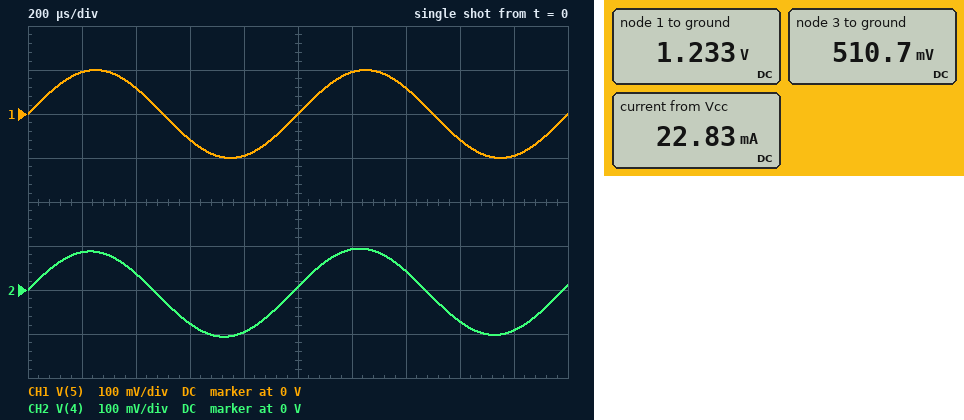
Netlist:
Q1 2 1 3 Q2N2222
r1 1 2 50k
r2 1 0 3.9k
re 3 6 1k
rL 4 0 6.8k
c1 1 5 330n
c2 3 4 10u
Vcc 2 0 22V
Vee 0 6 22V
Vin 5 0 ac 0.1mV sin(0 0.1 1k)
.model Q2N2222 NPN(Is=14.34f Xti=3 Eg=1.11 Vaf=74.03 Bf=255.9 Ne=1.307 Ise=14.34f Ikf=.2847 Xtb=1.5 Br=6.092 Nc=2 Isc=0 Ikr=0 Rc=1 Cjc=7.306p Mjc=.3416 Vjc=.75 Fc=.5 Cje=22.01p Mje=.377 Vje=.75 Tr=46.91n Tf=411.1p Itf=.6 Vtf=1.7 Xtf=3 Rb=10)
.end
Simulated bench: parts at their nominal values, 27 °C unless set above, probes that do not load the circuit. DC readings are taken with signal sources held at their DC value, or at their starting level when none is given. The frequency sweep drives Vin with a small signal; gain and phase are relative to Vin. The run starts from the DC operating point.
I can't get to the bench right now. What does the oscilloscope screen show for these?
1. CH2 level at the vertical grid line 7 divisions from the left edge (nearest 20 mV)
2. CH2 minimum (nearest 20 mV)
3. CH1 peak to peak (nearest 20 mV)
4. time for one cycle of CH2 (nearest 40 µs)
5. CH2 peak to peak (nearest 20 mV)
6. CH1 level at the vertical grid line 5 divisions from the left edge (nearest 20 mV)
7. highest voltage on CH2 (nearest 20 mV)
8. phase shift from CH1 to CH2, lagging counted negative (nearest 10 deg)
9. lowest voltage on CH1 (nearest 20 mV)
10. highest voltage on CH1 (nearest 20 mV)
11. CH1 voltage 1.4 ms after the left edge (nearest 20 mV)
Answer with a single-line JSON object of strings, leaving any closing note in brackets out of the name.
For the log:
{"CH2 level at the vertical grid line 7 divisions from the left edge": "40 mV", "CH2 minimum": "-100 mV", "CH1 peak to peak": "200 mV", "time for one cycle of CH2": "1.00 ms", "CH2 peak to peak": "200 mV", "CH1 level at the vertical grid line 5 divisions from the left edge": "0 V", "highest voltage on CH2": "100 mV", "phase shift from CH1 to CH2, lagging counted negative": "10 deg", "lowest voltage on CH1": "-100 mV", "highest voltage on CH1": "100 mV", "CH1 voltage 1.4 ms after the left edge": "60 mV"}
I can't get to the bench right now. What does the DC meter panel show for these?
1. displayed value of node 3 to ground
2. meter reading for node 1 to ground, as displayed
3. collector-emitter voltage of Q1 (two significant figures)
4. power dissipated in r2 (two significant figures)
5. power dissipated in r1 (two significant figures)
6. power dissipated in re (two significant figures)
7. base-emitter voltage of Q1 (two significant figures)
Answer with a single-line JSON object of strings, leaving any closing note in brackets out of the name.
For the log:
{"displayed value of node 3 to ground": "510.7 mV", "meter reading for node 1 to ground, as displayed": "1.233 V", "collector-emitter voltage of Q1": "21 V", "power dissipated in r2": "390 µW", "power dissipated in r1": "8.6 mW", "power dissipated in re": "510 mW", "base-emitter voltage of Q1": "720 mV"}
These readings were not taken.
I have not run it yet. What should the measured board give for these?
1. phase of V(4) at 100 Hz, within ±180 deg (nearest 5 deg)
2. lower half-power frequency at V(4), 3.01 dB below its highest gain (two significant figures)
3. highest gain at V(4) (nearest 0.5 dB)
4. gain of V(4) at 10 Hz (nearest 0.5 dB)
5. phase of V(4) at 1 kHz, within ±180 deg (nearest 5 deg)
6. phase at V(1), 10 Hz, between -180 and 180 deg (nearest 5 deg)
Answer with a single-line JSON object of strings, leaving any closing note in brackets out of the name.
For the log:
{"phase of V(4) at 100 Hz, within ±180 deg": "55 deg", "lower half-power frequency at V(4), 3.01 dB below its highest gain": "140 Hz", "highest gain at V(4)": "0 dB", "gain of V(4) at 10 Hz": "-23.0 dB", "phase of V(4) at 1 kHz, within ±180 deg": "10 deg", "phase at V(1), 10 Hz, between -180 and 180 deg": "85 deg"}
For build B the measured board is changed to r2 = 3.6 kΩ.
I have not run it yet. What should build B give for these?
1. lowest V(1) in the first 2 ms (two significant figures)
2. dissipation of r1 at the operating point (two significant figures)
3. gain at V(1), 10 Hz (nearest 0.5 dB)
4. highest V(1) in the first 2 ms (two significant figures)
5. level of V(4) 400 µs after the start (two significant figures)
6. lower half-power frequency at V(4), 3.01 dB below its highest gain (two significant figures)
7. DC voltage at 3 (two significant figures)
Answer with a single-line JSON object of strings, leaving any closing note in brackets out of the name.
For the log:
{"lowest V(1) in the first 2 ms": "1.0 V", "dissipation of r1 at the operating point": "8.7 mW", "gain at V(1), 10 Hz": "-23.5 dB", "highest V(1) in the first 2 ms": "1.2 V", "level of V(4) 400 µs after the start": "36 mV", "lower half-power frequency at V(4), 3.01 dB below its highest gain": "150 Hz", "DC voltage at 3": "420 mV"}
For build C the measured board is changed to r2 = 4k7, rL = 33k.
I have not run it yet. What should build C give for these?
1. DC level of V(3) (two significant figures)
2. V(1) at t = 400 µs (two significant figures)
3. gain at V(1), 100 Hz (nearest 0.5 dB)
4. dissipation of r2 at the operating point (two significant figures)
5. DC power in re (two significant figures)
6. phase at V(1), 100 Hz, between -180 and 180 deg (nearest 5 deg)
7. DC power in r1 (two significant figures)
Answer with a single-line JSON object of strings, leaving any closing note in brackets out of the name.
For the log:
{"DC level of V(3)": "740 mV", "V(1) at t = 400 µs": "1.5 V", "gain at V(1), 100 Hz": "-3.5 dB", "dissipation of r2 at the operating point": "450 µW", "DC power in re": "520 mW", "phase at V(1), 100 Hz, between -180 and 180 deg": "50 deg", "DC power in r1": "8.4 mW"}
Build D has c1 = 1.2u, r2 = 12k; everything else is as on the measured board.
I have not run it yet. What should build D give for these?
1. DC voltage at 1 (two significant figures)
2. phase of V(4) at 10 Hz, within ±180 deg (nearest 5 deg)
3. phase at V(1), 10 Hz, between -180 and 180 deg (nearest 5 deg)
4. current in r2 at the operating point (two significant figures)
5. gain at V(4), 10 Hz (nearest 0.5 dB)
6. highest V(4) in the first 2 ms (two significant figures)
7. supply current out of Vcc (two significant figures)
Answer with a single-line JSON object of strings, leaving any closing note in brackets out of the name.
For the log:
{"DC voltage at 1": "3.2 V", "phase of V(4) at 10 Hz, within ±180 deg": "70 deg", "phase at V(1), 10 Hz, between -180 and 180 deg": "55 deg", "current in r2 at the operating point": "270 µA", "gain at V(4), 10 Hz": "-5.0 dB", "highest V(4) in the first 2 ms": "98 mV", "supply current out of Vcc": "25 mA"}
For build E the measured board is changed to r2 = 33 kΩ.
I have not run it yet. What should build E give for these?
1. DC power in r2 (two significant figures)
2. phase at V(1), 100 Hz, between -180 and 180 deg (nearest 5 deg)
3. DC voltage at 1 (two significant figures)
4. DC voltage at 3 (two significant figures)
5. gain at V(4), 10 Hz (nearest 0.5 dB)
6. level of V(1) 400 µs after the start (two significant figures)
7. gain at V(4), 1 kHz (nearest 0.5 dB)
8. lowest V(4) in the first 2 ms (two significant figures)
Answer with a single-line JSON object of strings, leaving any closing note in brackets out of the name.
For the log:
{"DC power in r2": "1.2 mW", "phase at V(1), 100 Hz, between -180 and 180 deg": "15 deg", "DC voltage at 1": "6.2 V", "DC voltage at 3": "5.5 V", "gain at V(4), 10 Hz": "-9.5 dB", "level of V(1) 400 µs after the start": "6.3 V", "gain at V(4), 1 kHz": "0 dB", "lowest V(4) in the first 2 ms": "-100 mV"}
